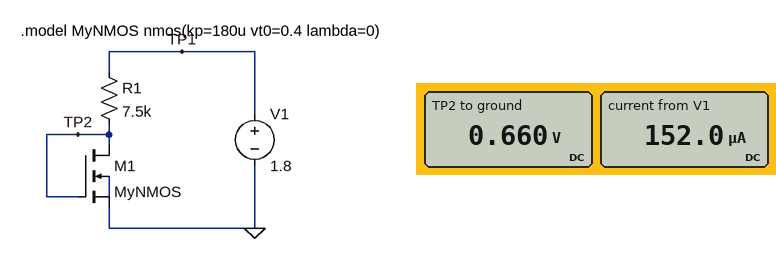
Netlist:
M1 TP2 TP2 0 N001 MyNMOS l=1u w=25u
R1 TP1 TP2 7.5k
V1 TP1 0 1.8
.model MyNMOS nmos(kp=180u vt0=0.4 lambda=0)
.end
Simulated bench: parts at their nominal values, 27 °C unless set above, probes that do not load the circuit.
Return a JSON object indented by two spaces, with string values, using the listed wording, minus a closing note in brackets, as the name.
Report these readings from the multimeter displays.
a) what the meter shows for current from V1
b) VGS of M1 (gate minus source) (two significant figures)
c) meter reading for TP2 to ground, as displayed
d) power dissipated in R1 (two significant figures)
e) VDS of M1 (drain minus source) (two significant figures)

{
  "what the meter shows for current from V1": "152.0 µA",
  "VGS of M1 (gate minus source)": "660 mV",
  "meter reading for TP2 to ground, as displayed": "0.660 V",
  "power dissipated in R1": "170 µW",
  "VDS of M1 (drain minus source)": "660 mV"
}
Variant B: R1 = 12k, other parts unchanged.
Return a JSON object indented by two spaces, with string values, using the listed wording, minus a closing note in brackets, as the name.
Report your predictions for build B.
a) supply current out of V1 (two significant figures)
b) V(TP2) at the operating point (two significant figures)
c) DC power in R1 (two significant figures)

{
  "supply current out of V1": "99 µA",
  "V(TP2) at the operating point": "610 mV",
  "DC power in R1": "120 µW"
}
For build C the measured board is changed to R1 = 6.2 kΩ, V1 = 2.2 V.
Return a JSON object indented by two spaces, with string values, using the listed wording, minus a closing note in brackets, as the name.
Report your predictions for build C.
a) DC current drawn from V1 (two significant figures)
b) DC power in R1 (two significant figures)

{
  "DC current drawn from V1": "240 µA",
  "DC power in R1": "350 µW"
}
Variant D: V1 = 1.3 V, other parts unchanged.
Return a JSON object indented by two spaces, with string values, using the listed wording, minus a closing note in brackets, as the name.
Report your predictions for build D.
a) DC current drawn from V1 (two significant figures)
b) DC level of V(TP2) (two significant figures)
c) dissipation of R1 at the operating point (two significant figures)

{
  "DC current drawn from V1": "93 µA",
  "DC level of V(TP2)": "600 mV",
  "dissipation of R1 at the operating point": "65 µW"
}
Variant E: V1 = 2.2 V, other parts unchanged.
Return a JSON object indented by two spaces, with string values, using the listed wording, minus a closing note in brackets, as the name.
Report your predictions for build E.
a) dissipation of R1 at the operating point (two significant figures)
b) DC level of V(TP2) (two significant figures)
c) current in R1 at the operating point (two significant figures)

{
  "dissipation of R1 at the operating point": "300 µW",
  "DC level of V(TP2)": "700 mV",
  "current in R1 at the operating point": "200 µA"
}
